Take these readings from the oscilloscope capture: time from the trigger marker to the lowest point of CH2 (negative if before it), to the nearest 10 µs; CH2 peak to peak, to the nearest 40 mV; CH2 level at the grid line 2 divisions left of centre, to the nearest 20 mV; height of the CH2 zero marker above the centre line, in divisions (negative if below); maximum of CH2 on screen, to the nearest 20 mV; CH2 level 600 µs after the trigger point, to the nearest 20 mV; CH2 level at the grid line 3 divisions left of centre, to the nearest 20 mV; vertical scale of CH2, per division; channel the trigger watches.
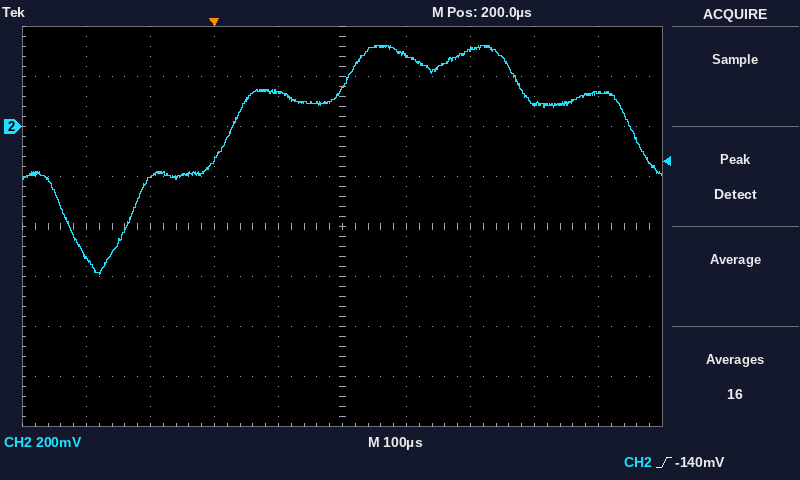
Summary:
-180 µs
920 mV
-140 mV
+2.0 div
320 mV
140 mV
-200 mV
200 mV
CH2
